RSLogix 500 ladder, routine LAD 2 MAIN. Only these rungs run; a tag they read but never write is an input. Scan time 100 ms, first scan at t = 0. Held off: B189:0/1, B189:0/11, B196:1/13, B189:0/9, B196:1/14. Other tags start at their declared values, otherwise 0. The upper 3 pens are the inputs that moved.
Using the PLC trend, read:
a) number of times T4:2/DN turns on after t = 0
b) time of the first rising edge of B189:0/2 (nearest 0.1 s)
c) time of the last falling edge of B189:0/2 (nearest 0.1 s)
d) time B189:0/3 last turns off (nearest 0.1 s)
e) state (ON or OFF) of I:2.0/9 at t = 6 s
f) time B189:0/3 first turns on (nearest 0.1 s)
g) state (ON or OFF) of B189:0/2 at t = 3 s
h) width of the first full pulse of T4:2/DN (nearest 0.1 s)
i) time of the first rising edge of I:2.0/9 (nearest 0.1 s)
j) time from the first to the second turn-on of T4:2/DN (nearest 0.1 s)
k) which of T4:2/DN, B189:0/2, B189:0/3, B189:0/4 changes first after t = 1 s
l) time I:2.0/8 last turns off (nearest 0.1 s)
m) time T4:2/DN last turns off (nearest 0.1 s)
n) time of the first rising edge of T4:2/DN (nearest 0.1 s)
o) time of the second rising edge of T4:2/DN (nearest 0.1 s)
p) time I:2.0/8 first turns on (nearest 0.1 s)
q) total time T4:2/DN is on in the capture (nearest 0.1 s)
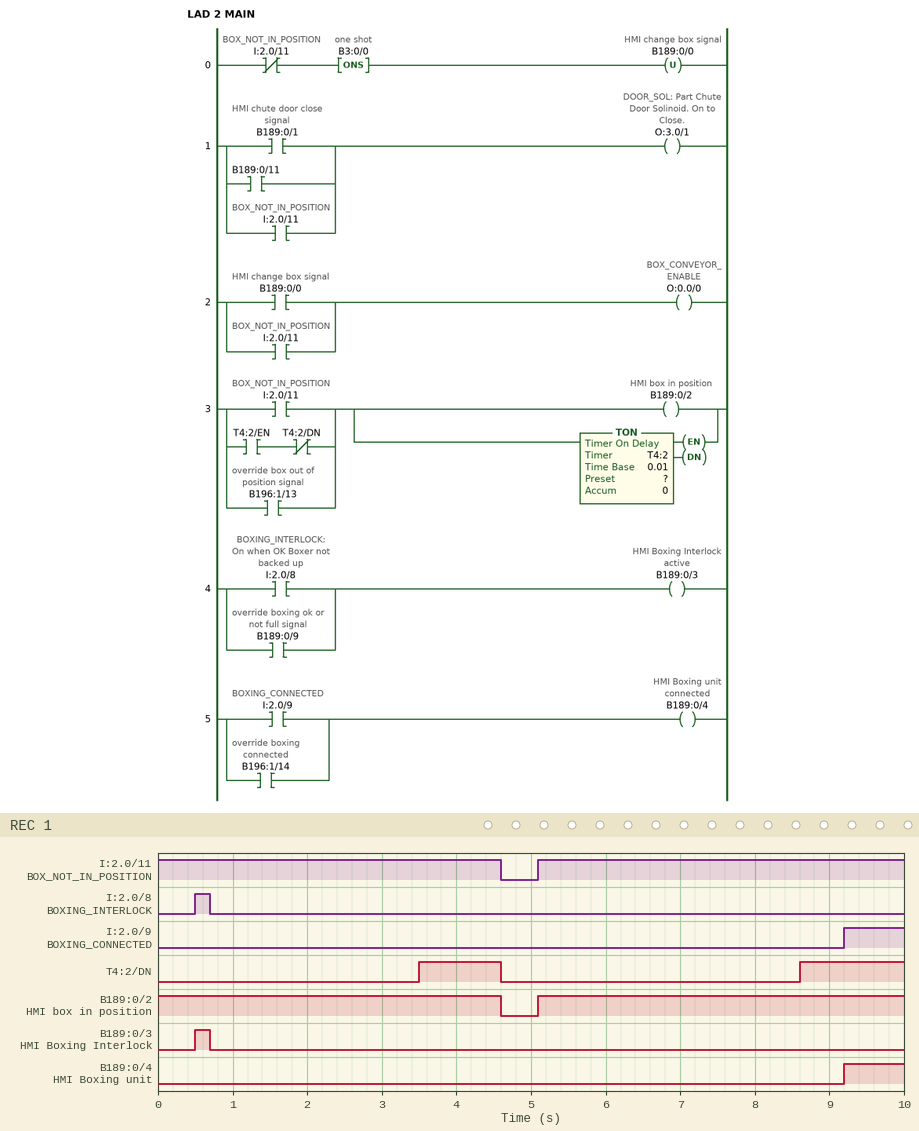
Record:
2
5.1 s
4.6 s
0.7 s
OFF
0.5 s
ON
1.1 s
9.2 s
5.1 s
T4:2/DN
0.7 s
4.6 s
3.5 s
8.6 s
0.5 s
2.5 s
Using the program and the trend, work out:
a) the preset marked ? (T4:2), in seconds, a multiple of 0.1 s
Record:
3.5 s
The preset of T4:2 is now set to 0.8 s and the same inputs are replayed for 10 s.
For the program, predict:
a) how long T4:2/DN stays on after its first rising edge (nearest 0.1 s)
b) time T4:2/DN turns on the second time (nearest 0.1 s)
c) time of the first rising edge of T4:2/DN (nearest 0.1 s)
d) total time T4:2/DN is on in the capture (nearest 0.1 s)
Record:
3.8 s
5.9 s
0.8 s
7.9 s
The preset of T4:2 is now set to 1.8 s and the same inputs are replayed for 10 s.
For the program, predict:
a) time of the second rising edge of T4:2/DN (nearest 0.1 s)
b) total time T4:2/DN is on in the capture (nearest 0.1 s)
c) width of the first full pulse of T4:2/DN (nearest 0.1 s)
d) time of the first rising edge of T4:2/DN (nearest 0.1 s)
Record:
6.9 s
5.9 s
2.8 s
1.8 s
